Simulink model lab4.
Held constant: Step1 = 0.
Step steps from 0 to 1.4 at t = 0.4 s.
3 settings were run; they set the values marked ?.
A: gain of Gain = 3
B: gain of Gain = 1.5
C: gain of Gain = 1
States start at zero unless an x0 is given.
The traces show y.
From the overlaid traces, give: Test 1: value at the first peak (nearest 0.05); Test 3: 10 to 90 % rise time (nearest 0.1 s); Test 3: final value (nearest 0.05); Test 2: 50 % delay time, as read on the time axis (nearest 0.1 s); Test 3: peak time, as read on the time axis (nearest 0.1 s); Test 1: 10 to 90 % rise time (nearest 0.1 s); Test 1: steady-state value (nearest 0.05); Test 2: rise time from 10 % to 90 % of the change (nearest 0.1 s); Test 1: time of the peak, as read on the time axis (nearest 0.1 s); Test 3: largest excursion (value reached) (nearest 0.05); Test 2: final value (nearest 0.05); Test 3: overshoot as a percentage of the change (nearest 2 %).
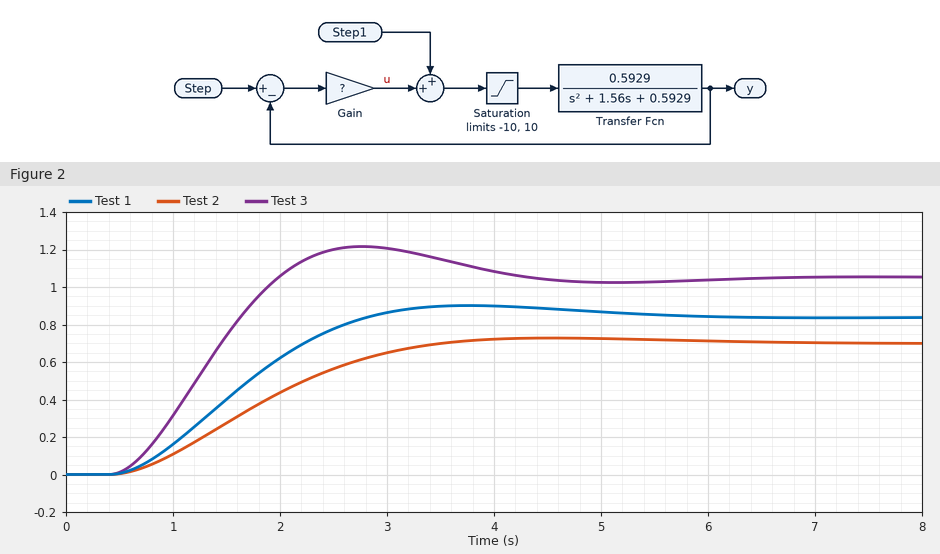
0.90
1.1 s
1.05
1.7 s
2.8 s
1.6 s
0.85
2.0 s
3.8 s
1.20
0.70
16 %
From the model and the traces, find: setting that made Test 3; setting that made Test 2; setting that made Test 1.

A
C
B
